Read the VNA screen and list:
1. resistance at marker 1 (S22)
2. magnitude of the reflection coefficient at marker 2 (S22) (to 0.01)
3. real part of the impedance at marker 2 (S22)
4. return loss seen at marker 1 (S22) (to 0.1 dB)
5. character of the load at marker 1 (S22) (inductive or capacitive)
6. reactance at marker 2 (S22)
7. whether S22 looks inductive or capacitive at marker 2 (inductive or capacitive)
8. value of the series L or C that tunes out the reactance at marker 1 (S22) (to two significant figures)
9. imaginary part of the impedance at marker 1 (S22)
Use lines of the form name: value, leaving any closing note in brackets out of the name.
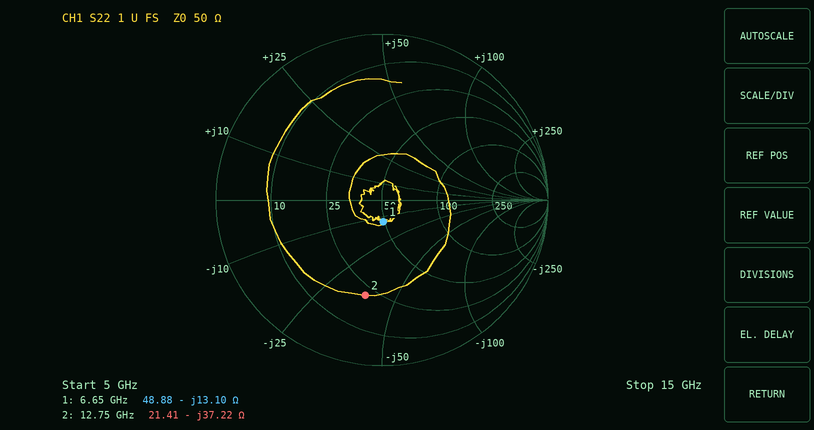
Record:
resistance at marker 1: 48.88 Ω
magnitude of the reflection coefficient at marker 2 (S22): 0.58
real part of the impedance at marker 2: 21.41 Ω
return loss seen at marker 1 (S22): 17.6 dB
character of the load at marker 1 (S22): capacitive
reactance at marker 2: -37.22 Ω
whether S22 looks inductive or capacitive at marker 2: capacitive
value of the series L or C that tunes out the reactance at marker 1 (S22): 310 pH
imaginary part of the impedance at marker 1: -13.10 Ω
